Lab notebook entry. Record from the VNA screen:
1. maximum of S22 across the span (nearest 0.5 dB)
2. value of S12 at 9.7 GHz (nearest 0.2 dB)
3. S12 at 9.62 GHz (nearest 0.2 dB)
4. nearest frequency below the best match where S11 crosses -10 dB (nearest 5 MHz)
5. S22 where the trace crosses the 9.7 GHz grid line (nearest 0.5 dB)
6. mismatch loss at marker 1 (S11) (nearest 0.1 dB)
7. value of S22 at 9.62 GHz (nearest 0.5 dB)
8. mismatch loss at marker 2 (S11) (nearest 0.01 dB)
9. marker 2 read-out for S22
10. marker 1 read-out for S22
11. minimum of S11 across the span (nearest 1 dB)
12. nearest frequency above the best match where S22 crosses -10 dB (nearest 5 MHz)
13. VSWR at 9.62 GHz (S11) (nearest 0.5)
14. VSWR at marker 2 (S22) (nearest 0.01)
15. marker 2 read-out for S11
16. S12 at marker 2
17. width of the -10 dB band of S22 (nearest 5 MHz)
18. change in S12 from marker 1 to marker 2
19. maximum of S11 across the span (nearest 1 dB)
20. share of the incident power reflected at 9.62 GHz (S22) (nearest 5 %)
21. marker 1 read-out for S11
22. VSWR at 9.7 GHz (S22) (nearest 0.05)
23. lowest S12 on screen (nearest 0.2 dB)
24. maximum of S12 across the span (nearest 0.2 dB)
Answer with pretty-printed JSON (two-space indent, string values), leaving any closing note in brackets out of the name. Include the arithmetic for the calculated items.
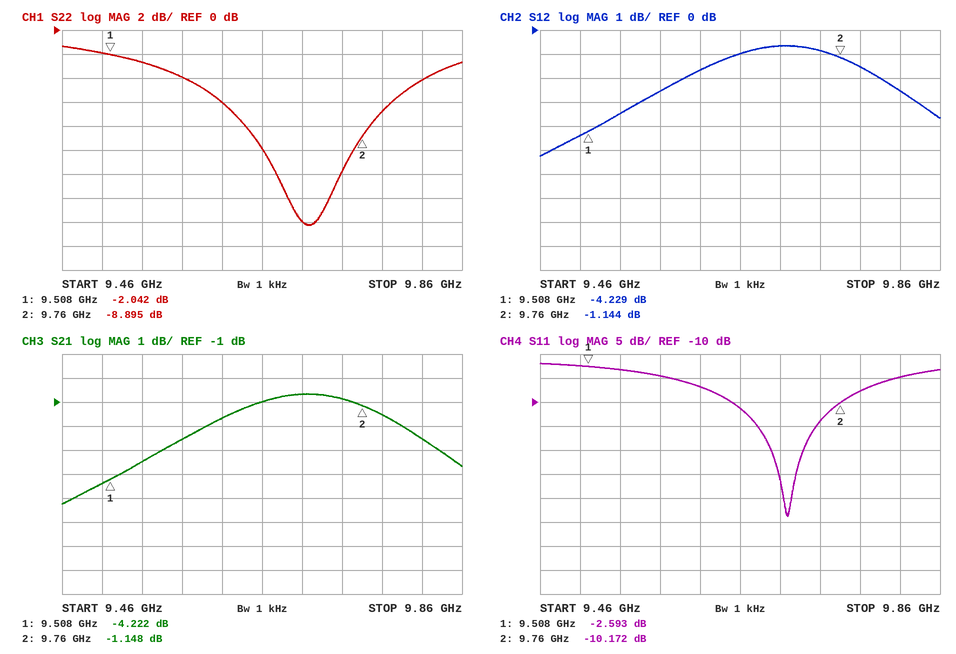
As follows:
{
  "maximum of S22 across the span": "-1.5 dB",
  "value of S12 at 9.7 GHz": "-0.6 dB",
  "S12 at 9.62 GHz": "-1.6 dB",
  "nearest frequency below the best match where S11 crosses -10 dB": "9.650 GHz",
  "S22 where the trace crosses the 9.7 GHz grid line": "-16.0 dB",
  "mismatch loss at marker 1 (S11)": "−10 log10(1 − 10^(-2.593/10)) ≈ 3.5 dB",
  "value of S22 at 9.62 GHz": "-6.0 dB",
  "mismatch loss at marker 2 (S11)": "−10 log10(1 − 10^(-10.172/10)) ≈ 0.44 dB",
  "marker 2 read-out for S22": "-8.895 dB",
  "marker 1 read-out for S22": "-2.042 dB",
  "minimum of S11 across the span": "-34 dB",
  "nearest frequency above the best match where S22 crosses -10 dB": "9.750 GHz",
  "VSWR at 9.62 GHz (S11)": "|Γ| = 10^(-7/20) = 0.4467; VSWR = (1 + 0.4467)/(1 − 0.4467) ≈ 2.61, so 2.5 to the nearest 0.5",
  "VSWR at marker 2 (S22)": "(1 + 0.3591)/(1 − 0.3591) ≈ 2.12",
  "marker 2 read-out for S11": "-10.172 dB",
  "S12 at marker 2": "-1.144 dB",
  "width of the -10 dB band of S22": "9.750 GHz − 9.660 GHz = 90 MHz",
  "change in S12 from marker 1 to marker 2": "-1.144 − (-4.229) = 3.085 dB",
  "maximum of S11 across the span": "-2 dB",
  "share of the incident power reflected at 9.62 GHz (S22)": "10^(-6/10) ≈ 25 %",
  "marker 1 read-out for S11": "-2.593 dB",
  "VSWR at 9.7 GHz (S22)": "|Γ| = 10^(-16/20) = 0.1585; VSWR = (1 + 0.1585)/(1 − 0.1585) ≈ 1.38, so 1.40 to the nearest 0.05",
  "lowest S12 on screen": "-5.2 dB",
  "maximum of S12 across the span": "-0.6 dB"
}
